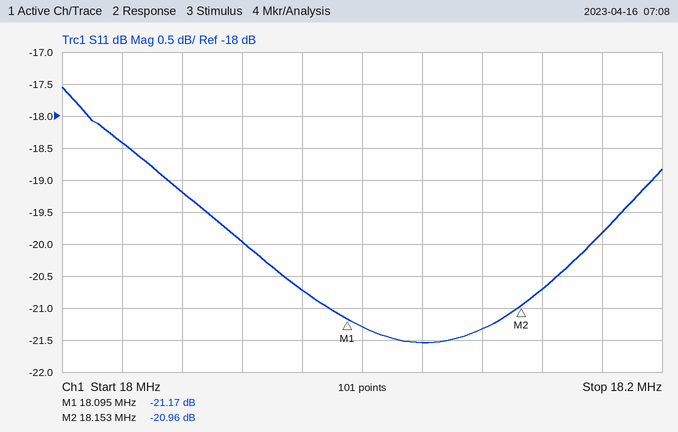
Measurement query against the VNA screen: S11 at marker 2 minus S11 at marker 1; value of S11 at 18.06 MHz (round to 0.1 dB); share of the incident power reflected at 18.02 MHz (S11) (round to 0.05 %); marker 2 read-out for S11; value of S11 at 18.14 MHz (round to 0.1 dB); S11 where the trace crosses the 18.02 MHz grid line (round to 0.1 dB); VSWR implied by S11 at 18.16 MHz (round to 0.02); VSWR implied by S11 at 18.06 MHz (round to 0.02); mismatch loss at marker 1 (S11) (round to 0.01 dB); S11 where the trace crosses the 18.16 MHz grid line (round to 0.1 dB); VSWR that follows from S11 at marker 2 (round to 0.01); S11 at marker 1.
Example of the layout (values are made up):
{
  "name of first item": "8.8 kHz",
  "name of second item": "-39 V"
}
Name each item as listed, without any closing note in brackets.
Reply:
{
  "S11 at marker 2 minus S11 at marker 1": "0.21 dB",
  "value of S11 at 18.06 MHz": "-20.0 dB",
  "share of the incident power reflected at 18.02 MHz (S11)": "1.45 %",
  "marker 2 read-out for S11": "-20.96 dB",
  "value of S11 at 18.14 MHz": "-21.3 dB",
  "S11 where the trace crosses the 18.02 MHz grid line": "-18.4 dB",
  "VSWR implied by S11 at 18.16 MHz": "1.20",
  "VSWR implied by S11 at 18.06 MHz": "1.22",
  "mismatch loss at marker 1 (S11)": "0.03 dB",
  "S11 where the trace crosses the 18.16 MHz grid line": "-20.7 dB",
  "VSWR that follows from S11 at marker 2": "1.20",
  "S11 at marker 1": "-21.17 dB"
}
